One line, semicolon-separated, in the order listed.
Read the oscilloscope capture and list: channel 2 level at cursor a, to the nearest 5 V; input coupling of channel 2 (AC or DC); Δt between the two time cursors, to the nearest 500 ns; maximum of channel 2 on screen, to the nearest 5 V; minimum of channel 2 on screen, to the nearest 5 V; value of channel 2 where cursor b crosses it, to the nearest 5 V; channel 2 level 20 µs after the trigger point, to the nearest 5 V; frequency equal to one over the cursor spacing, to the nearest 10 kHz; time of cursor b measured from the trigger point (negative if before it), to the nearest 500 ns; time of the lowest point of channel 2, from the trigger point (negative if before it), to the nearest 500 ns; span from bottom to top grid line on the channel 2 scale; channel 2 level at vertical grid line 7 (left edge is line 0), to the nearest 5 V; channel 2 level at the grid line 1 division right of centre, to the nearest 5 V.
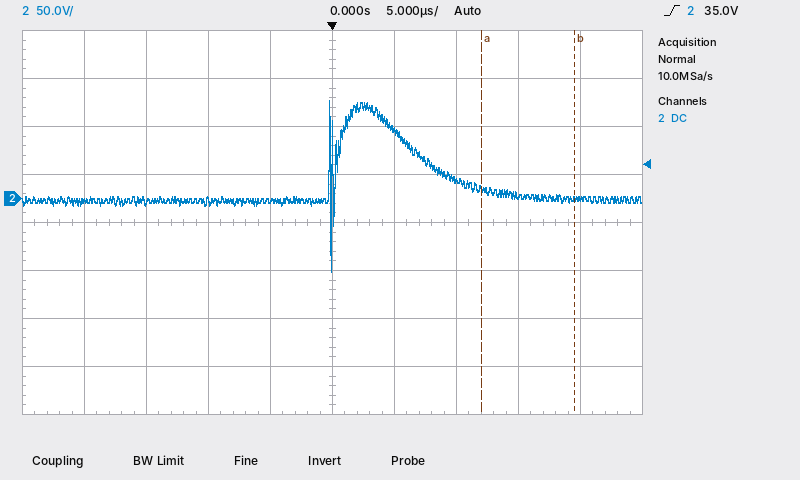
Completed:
10 V; DC; 7.5 µs; 100 V; -75 V; 0 V; 0 V; 130 kHz; +19.5 µs; 0.0 µs; 400 V; 20 V; 70 V
